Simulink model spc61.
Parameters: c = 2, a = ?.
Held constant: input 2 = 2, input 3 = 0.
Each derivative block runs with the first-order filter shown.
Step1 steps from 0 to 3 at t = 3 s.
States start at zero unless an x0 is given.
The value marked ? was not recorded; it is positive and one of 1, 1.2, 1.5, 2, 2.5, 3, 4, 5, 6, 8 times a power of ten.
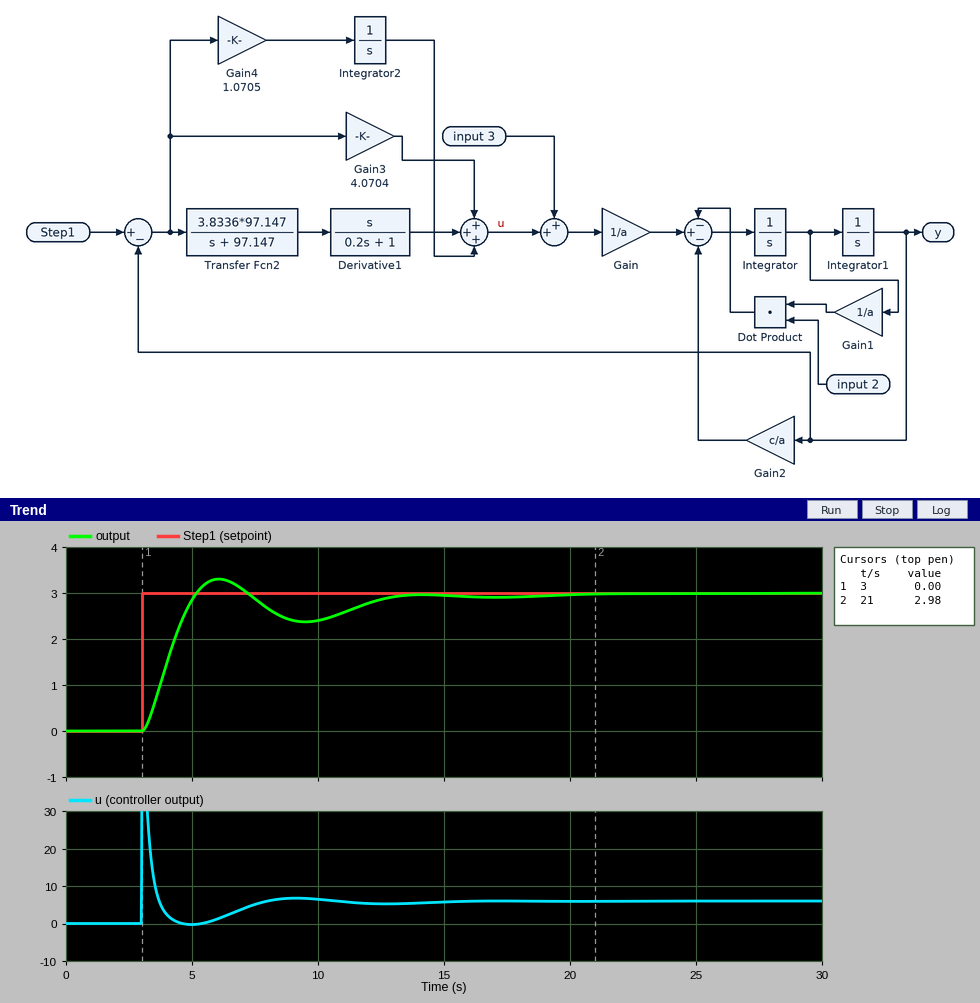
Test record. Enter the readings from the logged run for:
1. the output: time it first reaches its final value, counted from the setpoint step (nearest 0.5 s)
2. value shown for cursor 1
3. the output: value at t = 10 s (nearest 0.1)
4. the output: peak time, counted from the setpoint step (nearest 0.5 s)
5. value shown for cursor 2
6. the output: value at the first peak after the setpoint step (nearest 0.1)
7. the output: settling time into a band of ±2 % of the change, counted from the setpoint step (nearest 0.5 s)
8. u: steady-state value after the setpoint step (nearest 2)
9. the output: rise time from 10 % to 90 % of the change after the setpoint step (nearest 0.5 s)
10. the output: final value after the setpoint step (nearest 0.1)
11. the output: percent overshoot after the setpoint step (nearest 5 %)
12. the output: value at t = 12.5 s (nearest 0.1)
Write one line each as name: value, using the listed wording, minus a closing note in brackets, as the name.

the output: time it first reaches its final value, counted from the setpoint step: 2.0 s
value shown for cursor 1: 0.00
the output: value at t = 10 s: 2.4
the output: peak time, counted from the setpoint step: 3.0 s
value shown for cursor 2: 2.98
the output: value at the first peak after the setpoint step: 3.3
the output: settling time into a band of ±2 % of the change, counted from the setpoint step: 16.0 s
u: steady-state value after the setpoint step: 6
the output: rise time from 10 % to 90 % of the change after the setpoint step: 1.5 s
the output: final value after the setpoint step: 3.0
the output: percent overshoot after the setpoint step: 10 %
the output: value at t = 12.5 s: 2.9
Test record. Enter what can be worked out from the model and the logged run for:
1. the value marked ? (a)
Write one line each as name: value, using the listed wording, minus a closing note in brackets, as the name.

the value marked ?: 8
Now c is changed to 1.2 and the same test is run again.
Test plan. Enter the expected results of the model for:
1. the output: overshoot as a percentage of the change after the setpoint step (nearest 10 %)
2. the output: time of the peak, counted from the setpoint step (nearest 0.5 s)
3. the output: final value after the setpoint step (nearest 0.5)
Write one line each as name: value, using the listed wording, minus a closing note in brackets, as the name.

the output: overshoot as a percentage of the change after the setpoint step: 20 %
the output: time of the peak, counted from the setpoint step: 3.5 s
the output: final value after the setpoint step: 3.0
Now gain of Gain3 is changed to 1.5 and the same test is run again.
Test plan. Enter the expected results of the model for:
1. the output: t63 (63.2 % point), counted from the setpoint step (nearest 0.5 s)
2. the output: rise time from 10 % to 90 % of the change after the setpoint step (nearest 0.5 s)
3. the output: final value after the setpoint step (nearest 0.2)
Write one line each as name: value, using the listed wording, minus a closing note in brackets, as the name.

the output: t63 (63.2 % point), counted from the setpoint step: 1.5 s
the output: rise time from 10 % to 90 % of the change after the setpoint step: 2.5 s
the output: final value after the setpoint step: 3.0
